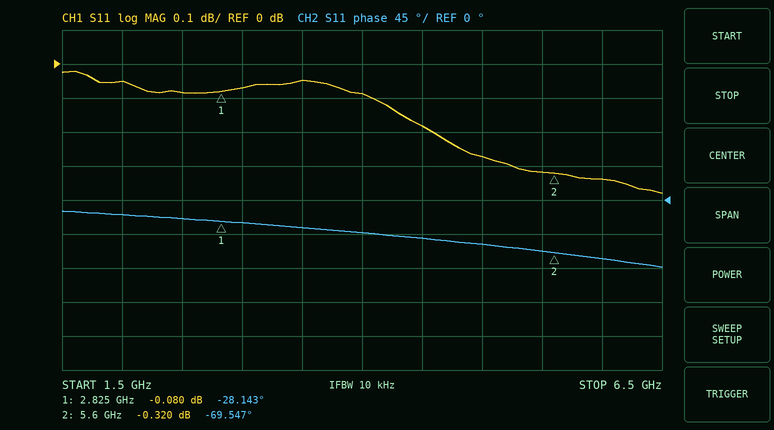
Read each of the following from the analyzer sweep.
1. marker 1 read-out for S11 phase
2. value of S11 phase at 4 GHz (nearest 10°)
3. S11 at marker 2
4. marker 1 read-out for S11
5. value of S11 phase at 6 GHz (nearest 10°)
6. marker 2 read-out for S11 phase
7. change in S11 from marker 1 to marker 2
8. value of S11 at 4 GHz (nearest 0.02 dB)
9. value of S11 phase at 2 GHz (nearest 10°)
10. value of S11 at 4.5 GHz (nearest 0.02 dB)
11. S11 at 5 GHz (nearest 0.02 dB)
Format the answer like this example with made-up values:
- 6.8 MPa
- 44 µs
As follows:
- -28.143°
- -40°
- -0.320 dB
- -0.080 dB
- -80°
- -69.547°
- -0.240 dB
- -0.08 dB
- -20°
- -0.18 dB
- -0.28 dB
